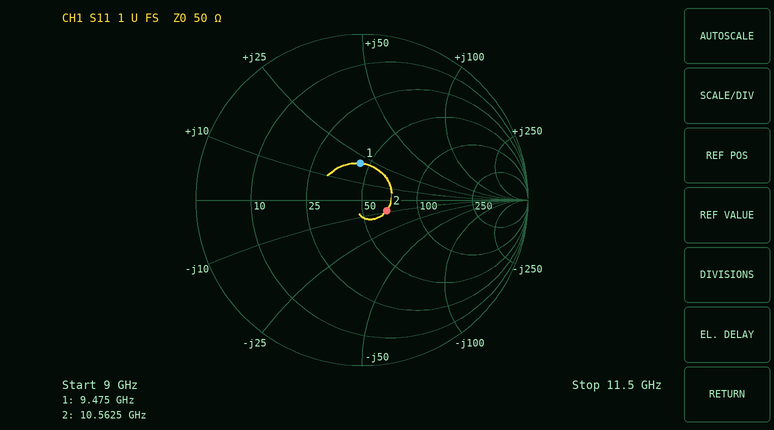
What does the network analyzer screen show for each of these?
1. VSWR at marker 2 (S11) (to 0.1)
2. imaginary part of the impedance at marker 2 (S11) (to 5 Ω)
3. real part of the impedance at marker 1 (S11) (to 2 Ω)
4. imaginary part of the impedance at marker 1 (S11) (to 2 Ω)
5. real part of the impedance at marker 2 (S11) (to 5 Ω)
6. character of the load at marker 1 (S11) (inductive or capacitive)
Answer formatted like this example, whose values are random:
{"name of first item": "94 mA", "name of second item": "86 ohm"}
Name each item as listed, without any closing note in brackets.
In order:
{"VSWR at marker 2 (S11)": "1.4", "imaginary part of the impedance at marker 2 (S11)": "-10 Ω", "real part of the impedance at marker 1 (S11)": "44 Ω", "imaginary part of the impedance at marker 1 (S11)": "+20 Ω", "real part of the impedance at marker 2 (S11)": "65 Ω", "character of the load at marker 1 (S11)": "inductive"}
